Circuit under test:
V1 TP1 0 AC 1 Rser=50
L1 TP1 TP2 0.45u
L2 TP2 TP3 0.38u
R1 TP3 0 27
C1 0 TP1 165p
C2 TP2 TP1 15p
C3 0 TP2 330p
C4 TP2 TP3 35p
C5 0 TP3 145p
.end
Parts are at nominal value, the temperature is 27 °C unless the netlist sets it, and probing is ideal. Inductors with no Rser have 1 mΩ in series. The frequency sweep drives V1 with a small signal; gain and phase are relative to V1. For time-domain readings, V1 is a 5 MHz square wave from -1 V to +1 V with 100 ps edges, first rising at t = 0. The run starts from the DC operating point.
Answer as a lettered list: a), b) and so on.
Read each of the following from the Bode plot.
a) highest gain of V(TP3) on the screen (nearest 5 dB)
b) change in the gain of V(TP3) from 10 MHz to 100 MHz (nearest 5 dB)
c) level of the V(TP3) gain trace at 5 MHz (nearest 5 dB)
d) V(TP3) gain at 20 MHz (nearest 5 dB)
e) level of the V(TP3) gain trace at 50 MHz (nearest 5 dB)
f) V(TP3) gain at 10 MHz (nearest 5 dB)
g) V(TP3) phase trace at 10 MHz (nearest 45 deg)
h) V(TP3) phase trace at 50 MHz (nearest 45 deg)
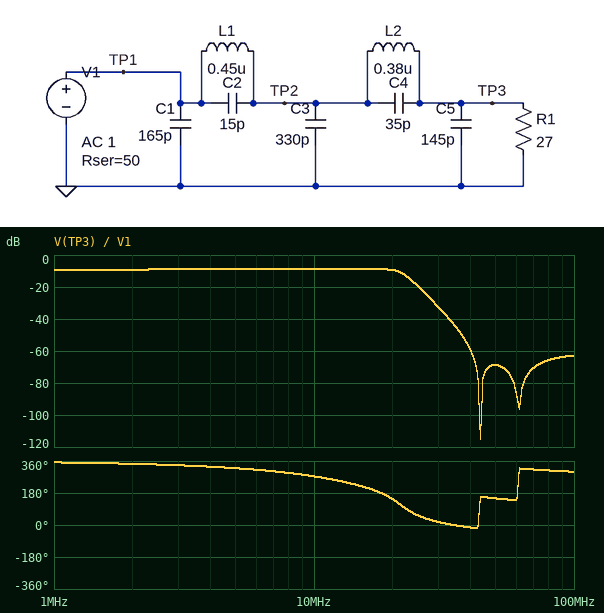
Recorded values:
a) -10 dB
b) -55 dB
c) -10 dB
d) -10 dB
e) -70 dB
f) -10 dB
g) 270 deg
h) 135 deg
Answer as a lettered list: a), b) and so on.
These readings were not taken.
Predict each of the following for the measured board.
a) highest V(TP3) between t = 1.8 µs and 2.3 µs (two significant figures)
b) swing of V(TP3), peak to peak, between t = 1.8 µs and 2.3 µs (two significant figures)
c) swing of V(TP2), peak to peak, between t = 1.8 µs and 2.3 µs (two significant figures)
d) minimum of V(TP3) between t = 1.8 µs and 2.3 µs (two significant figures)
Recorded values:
a) 480 mV
b) 960 mV
c) 1.3 V
d) -480 mV
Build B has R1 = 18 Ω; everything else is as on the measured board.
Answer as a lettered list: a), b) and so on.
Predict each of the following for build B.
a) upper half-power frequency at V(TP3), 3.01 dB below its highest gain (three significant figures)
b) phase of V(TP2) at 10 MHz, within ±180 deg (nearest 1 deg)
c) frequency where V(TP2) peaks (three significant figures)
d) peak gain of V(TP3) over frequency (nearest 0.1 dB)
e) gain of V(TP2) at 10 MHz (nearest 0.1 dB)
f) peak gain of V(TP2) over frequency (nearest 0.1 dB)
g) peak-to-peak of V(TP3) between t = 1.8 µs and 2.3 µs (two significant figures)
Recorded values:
a) 21.5 MHz
b) -25 deg
c) 19.9 MHz
d) -10.8 dB
e) -6.7 dB
f) -1.3 dB
g) 750 mV
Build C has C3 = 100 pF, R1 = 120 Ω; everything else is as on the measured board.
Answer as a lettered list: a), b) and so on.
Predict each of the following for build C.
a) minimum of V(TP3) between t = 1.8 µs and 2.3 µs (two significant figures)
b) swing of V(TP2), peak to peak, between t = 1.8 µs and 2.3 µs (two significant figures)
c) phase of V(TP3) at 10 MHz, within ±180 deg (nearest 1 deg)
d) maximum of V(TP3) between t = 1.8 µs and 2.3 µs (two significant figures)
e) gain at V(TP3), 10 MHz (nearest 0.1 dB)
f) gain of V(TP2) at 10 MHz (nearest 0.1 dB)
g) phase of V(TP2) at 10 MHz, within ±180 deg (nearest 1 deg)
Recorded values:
a) -920 mV
b) 1.7 V
c) -69 deg
d) 920 mV
e) -2.9 dB
f) -4.8 dB
g) -54 deg
